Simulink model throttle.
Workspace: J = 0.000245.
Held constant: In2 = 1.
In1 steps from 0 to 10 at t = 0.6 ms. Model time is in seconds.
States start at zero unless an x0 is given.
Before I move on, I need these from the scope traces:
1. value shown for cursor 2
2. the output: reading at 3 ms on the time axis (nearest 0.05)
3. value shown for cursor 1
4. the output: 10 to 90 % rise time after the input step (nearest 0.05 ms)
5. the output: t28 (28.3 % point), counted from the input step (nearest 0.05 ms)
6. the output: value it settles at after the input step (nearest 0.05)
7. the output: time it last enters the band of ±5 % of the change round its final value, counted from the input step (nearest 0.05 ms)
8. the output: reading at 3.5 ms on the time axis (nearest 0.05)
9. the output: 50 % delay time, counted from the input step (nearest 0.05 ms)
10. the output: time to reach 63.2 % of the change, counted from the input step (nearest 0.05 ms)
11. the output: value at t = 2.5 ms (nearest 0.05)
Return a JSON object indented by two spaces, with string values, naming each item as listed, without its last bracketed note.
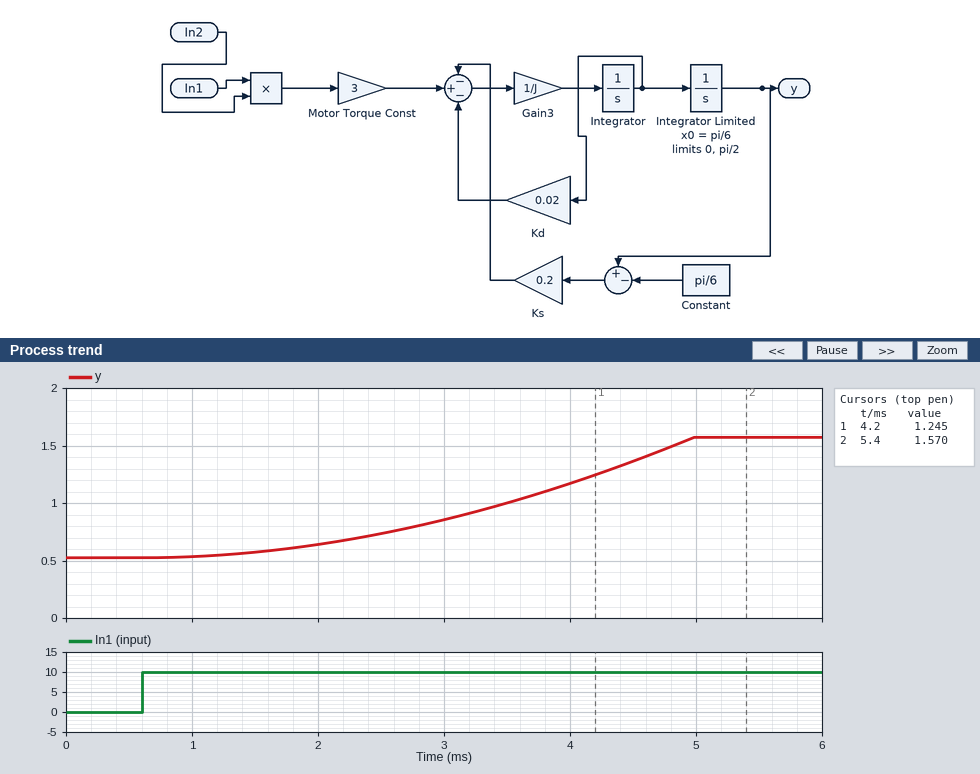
{
  "value shown for cursor 2": "1.570",
  "the output: reading at 3 ms on the time axis": "0.85",
  "value shown for cursor 1": "1.245",
  "the output: 10 to 90 % rise time after the input step": "2.80 ms",
  "the output: t28 (28.3 % point), counted from the input step": "2.25 ms",
  "the output: value it settles at after the input step": "1.55",
  "the output: time it last enters the band of ±5 % of the change round its final value, counted from the input step": "4.25 ms",
  "the output: reading at 3.5 ms on the time axis": "1.00",
  "the output: 50 % delay time, counted from the input step": "3.05 ms",
  "the output: time to reach 63.2 % of the change, counted from the input step": "3.45 ms",
  "the output: value at t = 2.5 ms": "0.75"
}
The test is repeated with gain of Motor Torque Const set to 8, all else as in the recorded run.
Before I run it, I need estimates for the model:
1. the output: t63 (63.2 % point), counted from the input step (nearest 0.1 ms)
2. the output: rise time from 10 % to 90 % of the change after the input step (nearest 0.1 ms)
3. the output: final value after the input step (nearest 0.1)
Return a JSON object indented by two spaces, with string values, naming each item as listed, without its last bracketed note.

{
  "the output: t63 (63.2 % point), counted from the input step": "2.1 ms",
  "the output: rise time from 10 % to 90 % of the change after the input step": "1.7 ms",
  "the output: final value after the input step": "1.6"
}
